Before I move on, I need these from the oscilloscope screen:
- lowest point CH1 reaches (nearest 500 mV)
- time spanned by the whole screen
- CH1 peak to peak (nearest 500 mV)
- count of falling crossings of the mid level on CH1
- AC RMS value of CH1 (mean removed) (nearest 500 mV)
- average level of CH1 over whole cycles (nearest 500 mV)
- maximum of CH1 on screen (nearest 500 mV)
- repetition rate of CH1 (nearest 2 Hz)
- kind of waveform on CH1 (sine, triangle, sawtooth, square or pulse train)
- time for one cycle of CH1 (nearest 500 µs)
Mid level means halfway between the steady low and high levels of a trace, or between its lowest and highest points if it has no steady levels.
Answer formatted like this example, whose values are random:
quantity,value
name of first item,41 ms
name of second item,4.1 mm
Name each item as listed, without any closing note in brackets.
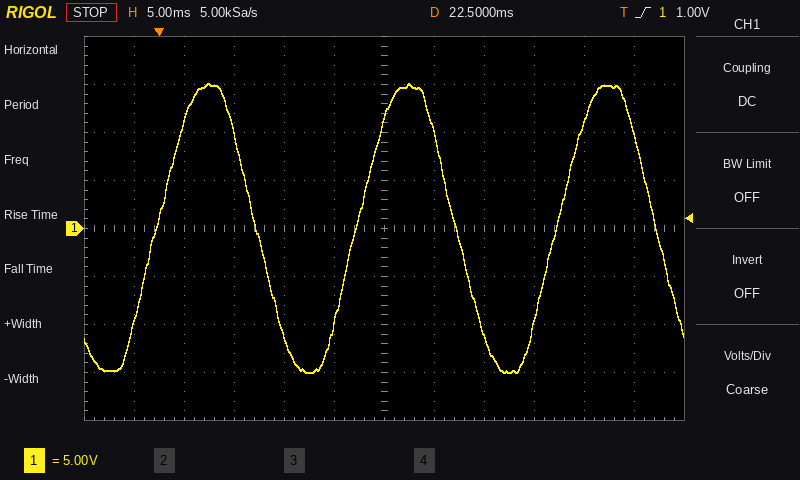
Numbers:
quantity,value
lowest point CH1 reaches,-15.0 V
time spanned by the whole screen,60 ms
CH1 peak to peak,30.0 V
count of falling crossings of the mid level on CH1,3
AC RMS value of CH1 (mean removed),10.5 V
average level of CH1 over whole cycles,0.0 V
maximum of CH1 on screen,15.0 V
repetition rate of CH1,50 Hz
kind of waveform on CH1,sine
time for one cycle of CH1,20.0 ms
